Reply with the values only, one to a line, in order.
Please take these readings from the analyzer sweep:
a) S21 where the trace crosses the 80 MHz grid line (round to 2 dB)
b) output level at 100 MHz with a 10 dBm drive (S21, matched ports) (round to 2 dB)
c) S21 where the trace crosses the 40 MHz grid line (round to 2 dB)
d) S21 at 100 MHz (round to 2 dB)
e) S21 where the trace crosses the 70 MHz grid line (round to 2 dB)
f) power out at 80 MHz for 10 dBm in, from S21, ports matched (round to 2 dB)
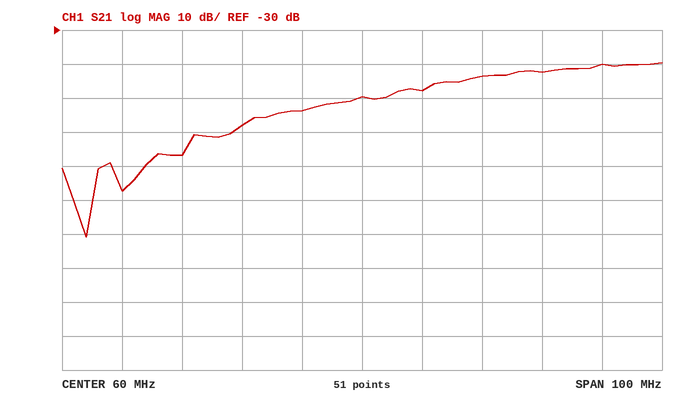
-44 dB
-30 dBm
-58 dB
-40 dB
-48 dB
-34 dBm
